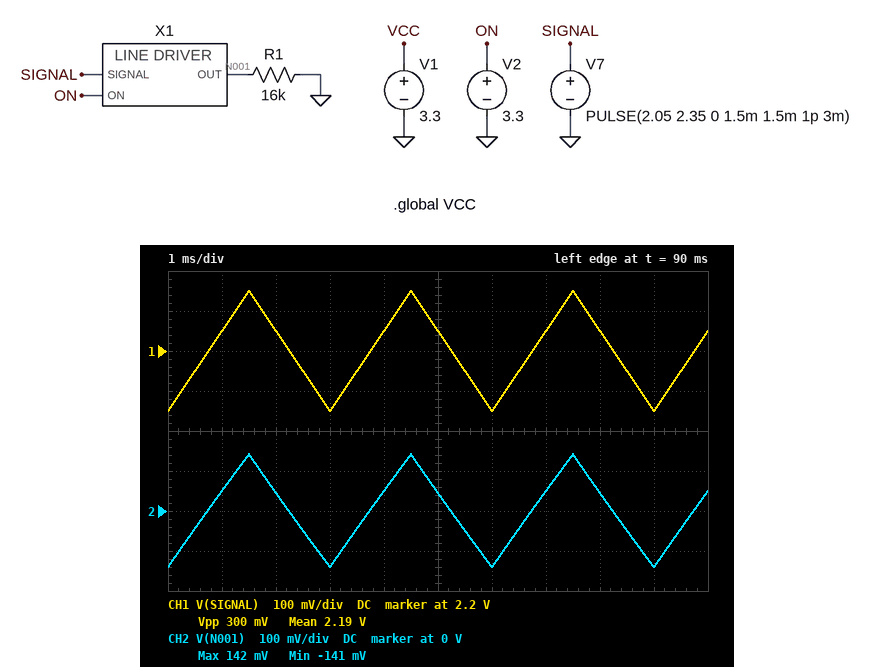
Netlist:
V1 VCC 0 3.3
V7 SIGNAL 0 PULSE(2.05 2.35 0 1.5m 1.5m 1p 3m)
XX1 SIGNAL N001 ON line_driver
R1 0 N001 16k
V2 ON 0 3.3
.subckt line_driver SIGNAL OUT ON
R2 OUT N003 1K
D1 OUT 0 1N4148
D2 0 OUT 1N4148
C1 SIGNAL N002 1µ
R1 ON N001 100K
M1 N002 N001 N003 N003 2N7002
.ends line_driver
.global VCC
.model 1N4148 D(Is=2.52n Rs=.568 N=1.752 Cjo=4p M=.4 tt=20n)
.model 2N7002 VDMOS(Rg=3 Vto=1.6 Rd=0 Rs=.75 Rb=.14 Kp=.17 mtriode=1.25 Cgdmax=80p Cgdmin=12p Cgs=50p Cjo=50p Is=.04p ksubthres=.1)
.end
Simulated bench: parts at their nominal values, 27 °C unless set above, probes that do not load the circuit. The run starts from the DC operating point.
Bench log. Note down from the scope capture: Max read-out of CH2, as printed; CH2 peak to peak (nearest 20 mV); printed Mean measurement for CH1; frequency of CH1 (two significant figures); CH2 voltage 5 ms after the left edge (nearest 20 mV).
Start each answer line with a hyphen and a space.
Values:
- 142 mV
- 280 mV
- 2.19 V
- 330 Hz
- 40 mV
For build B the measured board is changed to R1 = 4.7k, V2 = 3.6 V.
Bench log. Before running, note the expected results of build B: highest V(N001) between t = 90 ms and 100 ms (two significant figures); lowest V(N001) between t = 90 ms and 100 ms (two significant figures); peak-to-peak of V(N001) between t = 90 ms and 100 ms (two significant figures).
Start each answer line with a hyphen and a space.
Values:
- 120 mV
- -120 mV
- 250 mV
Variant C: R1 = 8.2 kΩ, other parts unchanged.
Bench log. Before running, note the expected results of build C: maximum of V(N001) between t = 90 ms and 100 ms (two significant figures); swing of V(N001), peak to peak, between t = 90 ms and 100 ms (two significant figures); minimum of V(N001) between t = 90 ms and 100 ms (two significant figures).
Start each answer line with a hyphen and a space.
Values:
- 130 mV
- 270 mV
- -130 mV
